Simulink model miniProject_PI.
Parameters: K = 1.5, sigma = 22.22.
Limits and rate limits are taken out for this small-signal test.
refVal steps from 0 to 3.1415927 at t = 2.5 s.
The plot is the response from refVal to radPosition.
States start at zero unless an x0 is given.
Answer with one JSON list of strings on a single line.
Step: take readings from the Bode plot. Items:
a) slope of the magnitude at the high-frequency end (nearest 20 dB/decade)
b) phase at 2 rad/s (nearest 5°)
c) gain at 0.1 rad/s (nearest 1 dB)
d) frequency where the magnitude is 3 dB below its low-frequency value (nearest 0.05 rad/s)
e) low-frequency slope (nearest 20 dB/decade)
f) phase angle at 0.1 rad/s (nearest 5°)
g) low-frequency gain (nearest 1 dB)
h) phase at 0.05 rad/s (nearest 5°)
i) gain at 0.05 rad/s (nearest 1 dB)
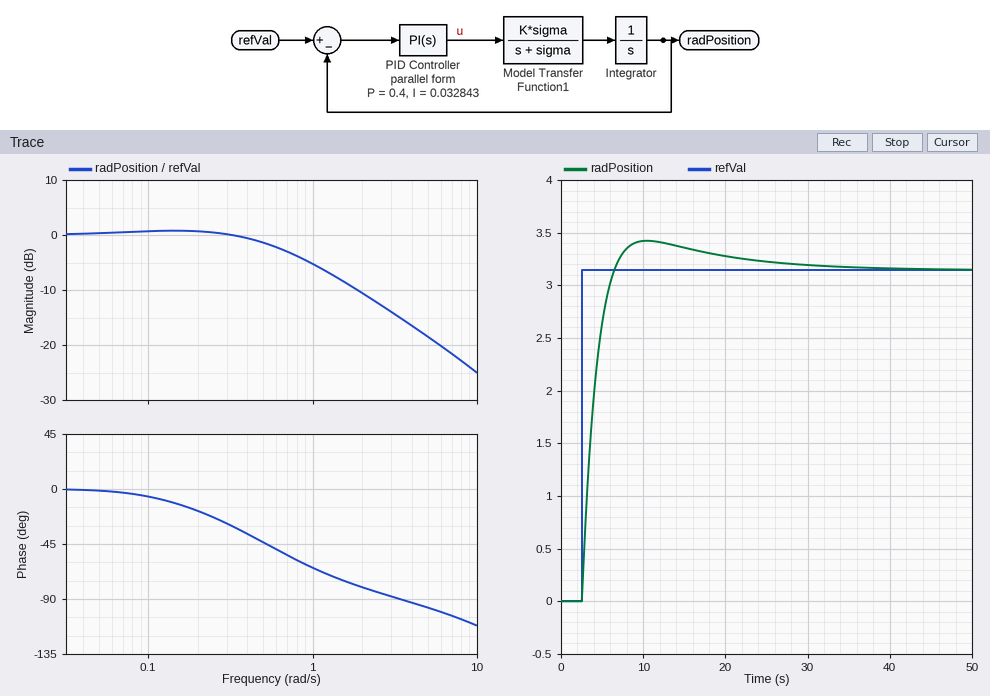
["-20 dB/decade", "-80°", "1 dB", "0.65 rad/s", "0 dB/decade", "-5°", "0 dB", "0°", "0 dB"]
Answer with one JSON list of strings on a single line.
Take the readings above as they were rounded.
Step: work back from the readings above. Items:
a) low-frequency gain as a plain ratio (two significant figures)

["1.0"]
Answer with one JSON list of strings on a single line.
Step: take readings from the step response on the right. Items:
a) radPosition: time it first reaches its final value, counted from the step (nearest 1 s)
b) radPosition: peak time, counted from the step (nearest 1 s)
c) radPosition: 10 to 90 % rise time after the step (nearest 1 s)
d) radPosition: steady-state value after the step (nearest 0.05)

["4 s", "8 s", "3 s", "3.15"]
